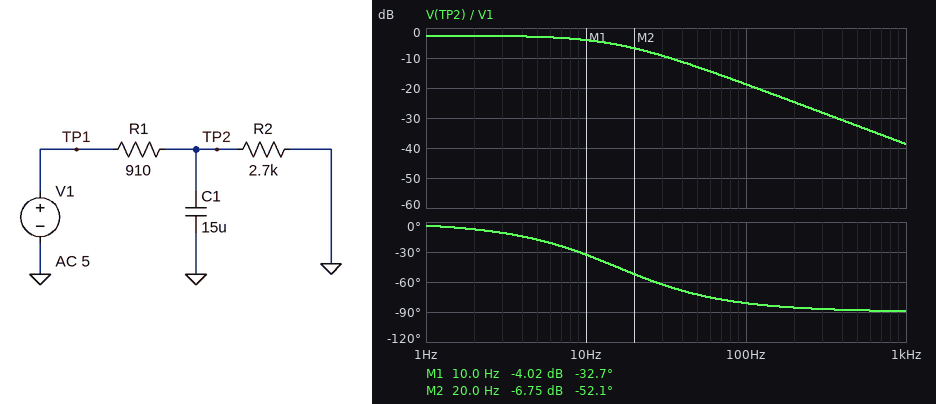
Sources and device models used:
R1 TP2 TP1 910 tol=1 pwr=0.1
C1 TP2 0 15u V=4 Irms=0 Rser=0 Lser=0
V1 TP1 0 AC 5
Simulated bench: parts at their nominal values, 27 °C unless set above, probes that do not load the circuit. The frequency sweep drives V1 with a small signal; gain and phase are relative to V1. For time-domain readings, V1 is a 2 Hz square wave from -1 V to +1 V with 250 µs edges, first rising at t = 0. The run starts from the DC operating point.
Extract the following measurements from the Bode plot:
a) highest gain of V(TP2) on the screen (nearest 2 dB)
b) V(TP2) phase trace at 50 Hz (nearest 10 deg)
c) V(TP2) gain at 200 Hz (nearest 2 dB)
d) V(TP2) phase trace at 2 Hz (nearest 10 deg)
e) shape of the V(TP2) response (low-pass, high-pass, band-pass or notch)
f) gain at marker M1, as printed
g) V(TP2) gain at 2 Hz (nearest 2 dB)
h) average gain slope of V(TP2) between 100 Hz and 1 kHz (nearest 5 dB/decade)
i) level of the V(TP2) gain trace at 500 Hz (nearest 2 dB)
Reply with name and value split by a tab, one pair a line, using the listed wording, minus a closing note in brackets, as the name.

highest gain of V(TP2) on the screen	-2 dB
V(TP2) phase trace at 50 Hz	-70 deg
V(TP2) gain at 200 Hz	-24 dB
V(TP2) phase trace at 2 Hz	-10 deg
shape of the V(TP2) response	low-pass
gain at marker M1, as printed	-4.02 dB
V(TP2) gain at 2 Hz	-2 dB
average gain slope of V(TP2) between 100 Hz and 1 kHz	-20 dB/decade
level of the V(TP2) gain trace at 500 Hz	-32 dB
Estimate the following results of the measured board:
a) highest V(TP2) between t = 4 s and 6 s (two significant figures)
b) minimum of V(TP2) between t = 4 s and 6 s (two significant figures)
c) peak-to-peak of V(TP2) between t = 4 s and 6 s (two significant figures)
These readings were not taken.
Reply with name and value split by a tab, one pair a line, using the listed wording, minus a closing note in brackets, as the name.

highest V(TP2) between t = 4 s and 6 s	750 mV
minimum of V(TP2) between t = 4 s and 6 s	-750 mV
peak-to-peak of V(TP2) between t = 4 s and 6 s	1.5 V
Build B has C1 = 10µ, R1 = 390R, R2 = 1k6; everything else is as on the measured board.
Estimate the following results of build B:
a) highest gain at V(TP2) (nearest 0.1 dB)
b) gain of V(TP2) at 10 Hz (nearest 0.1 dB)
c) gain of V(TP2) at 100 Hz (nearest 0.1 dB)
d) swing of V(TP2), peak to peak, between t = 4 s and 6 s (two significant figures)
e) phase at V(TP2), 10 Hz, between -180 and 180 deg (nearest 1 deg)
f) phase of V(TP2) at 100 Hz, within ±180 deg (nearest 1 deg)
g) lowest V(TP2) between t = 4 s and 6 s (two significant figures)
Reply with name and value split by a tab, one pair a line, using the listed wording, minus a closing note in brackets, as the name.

highest gain at V(TP2)	-1.9 dB
gain of V(TP2) at 10 Hz	-2.1 dB
gain of V(TP2) at 100 Hz	-8.8 dB
swing of V(TP2), peak to peak, between t = 4 s and 6 s	1.6 V
phase at V(TP2), 10 Hz, between -180 and 180 deg	-11 deg
phase of V(TP2) at 100 Hz, within ±180 deg	-63 deg
lowest V(TP2) between t = 4 s and 6 s	-800 mV
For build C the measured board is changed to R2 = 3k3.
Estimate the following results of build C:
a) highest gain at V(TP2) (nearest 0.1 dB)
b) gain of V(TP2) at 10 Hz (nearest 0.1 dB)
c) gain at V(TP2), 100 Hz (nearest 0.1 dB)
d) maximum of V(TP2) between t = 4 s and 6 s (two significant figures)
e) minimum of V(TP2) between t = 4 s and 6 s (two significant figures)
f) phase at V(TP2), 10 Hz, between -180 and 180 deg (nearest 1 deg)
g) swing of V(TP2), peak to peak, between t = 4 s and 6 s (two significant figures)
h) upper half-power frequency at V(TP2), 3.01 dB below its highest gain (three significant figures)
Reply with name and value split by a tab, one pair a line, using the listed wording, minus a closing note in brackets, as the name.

highest gain at V(TP2)	-2.1 dB
gain of V(TP2) at 10 Hz	-3.7 dB
gain at V(TP2), 100 Hz	-18.8 dB
maximum of V(TP2) between t = 4 s and 6 s	780 mV
minimum of V(TP2) between t = 4 s and 6 s	-780 mV
phase at V(TP2), 10 Hz, between -180 and 180 deg	-34 deg
swing of V(TP2), peak to peak, between t = 4 s and 6 s	1.6 V
upper half-power frequency at V(TP2), 3.01 dB below its highest gain	14.9 Hz
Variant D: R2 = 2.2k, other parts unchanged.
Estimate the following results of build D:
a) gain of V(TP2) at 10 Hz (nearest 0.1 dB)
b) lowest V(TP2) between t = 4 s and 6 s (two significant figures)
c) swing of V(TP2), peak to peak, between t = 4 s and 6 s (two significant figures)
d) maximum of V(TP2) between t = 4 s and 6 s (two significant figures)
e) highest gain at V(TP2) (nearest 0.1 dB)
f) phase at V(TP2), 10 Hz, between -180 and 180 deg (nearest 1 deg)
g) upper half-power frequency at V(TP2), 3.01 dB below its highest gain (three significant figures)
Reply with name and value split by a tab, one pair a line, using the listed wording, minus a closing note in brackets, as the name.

gain of V(TP2) at 10 Hz	-4.4 dB
lowest V(TP2) between t = 4 s and 6 s	-710 mV
swing of V(TP2), peak to peak, between t = 4 s and 6 s	1.4 V
maximum of V(TP2) between t = 4 s and 6 s	710 mV
highest gain at V(TP2)	-3.0 dB
phase at V(TP2), 10 Hz, between -180 and 180 deg	-31 deg
upper half-power frequency at V(TP2), 3.01 dB below its highest gain	16.5 Hz
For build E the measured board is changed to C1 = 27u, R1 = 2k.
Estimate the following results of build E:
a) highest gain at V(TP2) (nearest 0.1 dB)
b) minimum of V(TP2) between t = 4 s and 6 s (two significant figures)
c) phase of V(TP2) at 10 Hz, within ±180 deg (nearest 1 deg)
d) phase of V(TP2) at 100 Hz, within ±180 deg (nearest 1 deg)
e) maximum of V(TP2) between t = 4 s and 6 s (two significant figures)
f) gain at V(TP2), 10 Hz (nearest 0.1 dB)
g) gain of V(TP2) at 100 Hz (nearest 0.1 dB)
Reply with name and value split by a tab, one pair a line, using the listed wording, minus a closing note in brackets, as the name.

highest gain at V(TP2)	-4.8 dB
minimum of V(TP2) between t = 4 s and 6 s	-570 mV
phase of V(TP2) at 10 Hz, within ±180 deg	-63 deg
phase of V(TP2) at 100 Hz, within ±180 deg	-87 deg
maximum of V(TP2) between t = 4 s and 6 s	570 mV
gain at V(TP2), 10 Hz	-11.6 dB
gain of V(TP2) at 100 Hz	-30.6 dB
